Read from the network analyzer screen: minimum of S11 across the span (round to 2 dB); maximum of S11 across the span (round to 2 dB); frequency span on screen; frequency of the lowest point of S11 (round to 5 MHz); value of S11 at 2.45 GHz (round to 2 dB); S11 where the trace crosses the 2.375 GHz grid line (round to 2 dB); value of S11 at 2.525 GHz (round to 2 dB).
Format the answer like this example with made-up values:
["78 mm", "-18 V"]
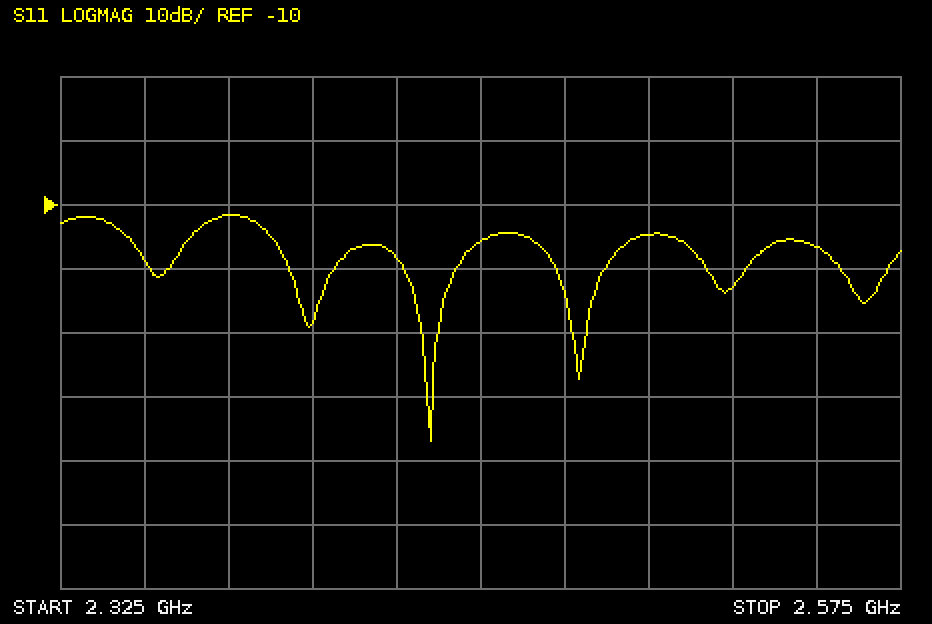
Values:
["-46 dB", "-12 dB", "250 MHz", "2.435 GHz", "-16 dB", "-12 dB", "-22 dB"]
